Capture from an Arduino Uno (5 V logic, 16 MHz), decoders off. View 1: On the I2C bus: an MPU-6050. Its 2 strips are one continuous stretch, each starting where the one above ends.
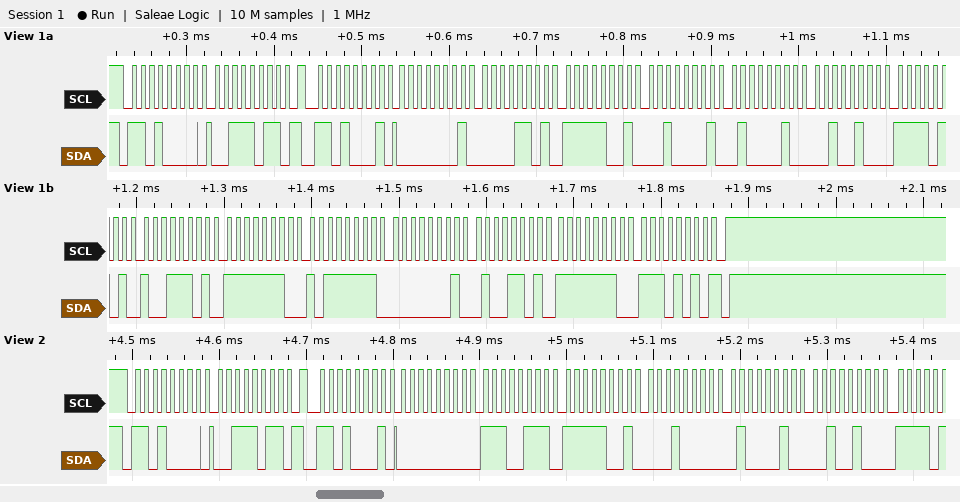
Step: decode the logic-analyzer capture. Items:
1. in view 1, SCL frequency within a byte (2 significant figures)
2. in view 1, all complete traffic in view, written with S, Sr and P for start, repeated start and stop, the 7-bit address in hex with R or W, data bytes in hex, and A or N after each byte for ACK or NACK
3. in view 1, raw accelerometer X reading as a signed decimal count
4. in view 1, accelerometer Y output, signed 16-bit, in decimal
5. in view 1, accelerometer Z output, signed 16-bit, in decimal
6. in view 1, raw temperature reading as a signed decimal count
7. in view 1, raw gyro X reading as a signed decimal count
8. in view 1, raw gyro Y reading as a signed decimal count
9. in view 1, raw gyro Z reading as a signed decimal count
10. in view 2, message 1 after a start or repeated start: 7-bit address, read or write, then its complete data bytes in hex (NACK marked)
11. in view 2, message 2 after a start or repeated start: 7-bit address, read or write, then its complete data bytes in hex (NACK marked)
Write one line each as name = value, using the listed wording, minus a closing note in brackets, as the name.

in view 1, SCL frequency within a byte = 100 kHz
in view 1, all complete traffic in view, written with S, Sr and P for start, repeated start and stop, the 7-bit address in hex with R or W, data bytes in hex, and A or N after each byte for ACK or NACK = S 68W A 3B A Sr 68R A 01 A 0D A F9 A 21 A 42 A 24 A F5 A 9D A FE A BF A 01 A 4D A FE A EA N P
in view 1, raw accelerometer X reading as a signed decimal count = 269
in view 1, accelerometer Y output, signed 16-bit, in decimal = -1759
in view 1, accelerometer Z output, signed 16-bit, in decimal = 16932
in view 1, raw temperature reading as a signed decimal count = -2659
in view 1, raw gyro X reading as a signed decimal count = -321
in view 1, raw gyro Y reading as a signed decimal count = 333
in view 1, raw gyro Z reading as a signed decimal count = -278
in view 2, message 1 after a start or repeated start: 7-bit address, read or write, then its complete data bytes in hex = 0x68 write: 3B
in view 2, message 2 after a start or repeated start: 7-bit address, read or write, then its complete data bytes in hex = 0x68 read: 00 E7 F9 10 42 24
